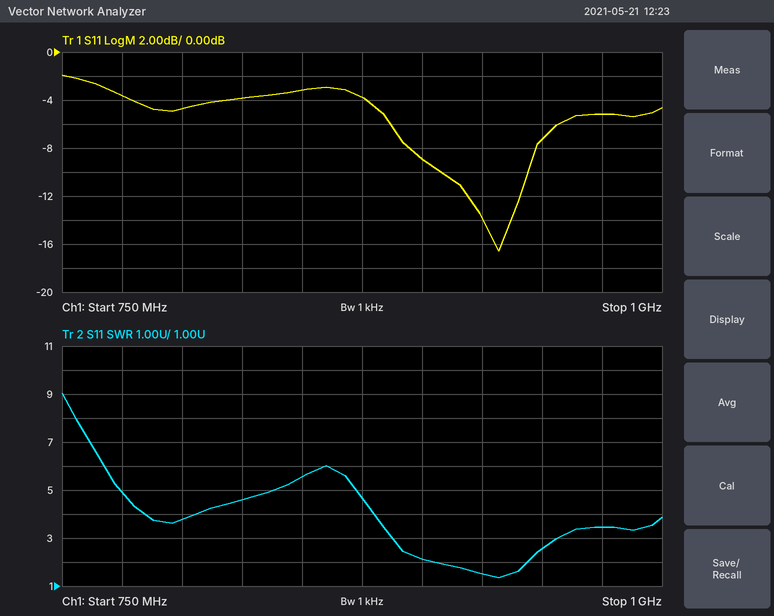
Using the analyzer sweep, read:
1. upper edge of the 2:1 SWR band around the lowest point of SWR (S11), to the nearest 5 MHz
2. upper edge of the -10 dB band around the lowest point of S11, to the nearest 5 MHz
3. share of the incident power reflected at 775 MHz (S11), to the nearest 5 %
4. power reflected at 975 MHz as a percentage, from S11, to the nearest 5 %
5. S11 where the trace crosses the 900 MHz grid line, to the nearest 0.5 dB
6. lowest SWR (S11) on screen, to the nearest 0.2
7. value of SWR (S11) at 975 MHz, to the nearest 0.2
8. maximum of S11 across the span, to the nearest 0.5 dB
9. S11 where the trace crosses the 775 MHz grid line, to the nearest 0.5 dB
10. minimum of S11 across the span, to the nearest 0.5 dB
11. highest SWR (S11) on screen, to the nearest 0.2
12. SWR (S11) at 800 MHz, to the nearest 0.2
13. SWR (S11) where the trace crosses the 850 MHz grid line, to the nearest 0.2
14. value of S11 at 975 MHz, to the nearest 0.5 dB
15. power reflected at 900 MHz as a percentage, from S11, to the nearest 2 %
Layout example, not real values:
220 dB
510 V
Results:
945 MHz
945 MHz
45 %
30 %
-9.0 dB
1.4
3.4
-2.0 dB
-3.5 dB
-16.5 dB
9.0
3.8
5.6
-5.0 dB
12 %
